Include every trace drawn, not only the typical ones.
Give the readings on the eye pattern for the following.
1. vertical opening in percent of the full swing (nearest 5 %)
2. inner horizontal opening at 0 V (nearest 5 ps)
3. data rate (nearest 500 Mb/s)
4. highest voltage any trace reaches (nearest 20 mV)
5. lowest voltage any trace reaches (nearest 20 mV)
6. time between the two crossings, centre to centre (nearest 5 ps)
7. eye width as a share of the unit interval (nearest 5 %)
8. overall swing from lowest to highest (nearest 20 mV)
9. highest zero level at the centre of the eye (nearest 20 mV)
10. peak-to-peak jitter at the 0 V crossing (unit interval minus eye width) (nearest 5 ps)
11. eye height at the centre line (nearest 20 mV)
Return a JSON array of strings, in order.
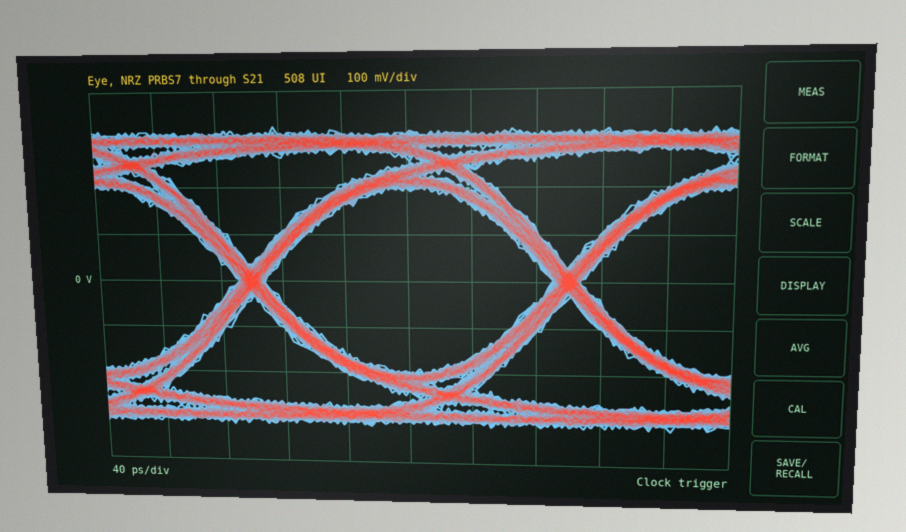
["60 %", "180 ps", "5.0 Gb/s", "320 mV", "-320 mV", "200 ps", "90 %", "640 mV", "-200 mV", "20 ps", "400 mV"]
